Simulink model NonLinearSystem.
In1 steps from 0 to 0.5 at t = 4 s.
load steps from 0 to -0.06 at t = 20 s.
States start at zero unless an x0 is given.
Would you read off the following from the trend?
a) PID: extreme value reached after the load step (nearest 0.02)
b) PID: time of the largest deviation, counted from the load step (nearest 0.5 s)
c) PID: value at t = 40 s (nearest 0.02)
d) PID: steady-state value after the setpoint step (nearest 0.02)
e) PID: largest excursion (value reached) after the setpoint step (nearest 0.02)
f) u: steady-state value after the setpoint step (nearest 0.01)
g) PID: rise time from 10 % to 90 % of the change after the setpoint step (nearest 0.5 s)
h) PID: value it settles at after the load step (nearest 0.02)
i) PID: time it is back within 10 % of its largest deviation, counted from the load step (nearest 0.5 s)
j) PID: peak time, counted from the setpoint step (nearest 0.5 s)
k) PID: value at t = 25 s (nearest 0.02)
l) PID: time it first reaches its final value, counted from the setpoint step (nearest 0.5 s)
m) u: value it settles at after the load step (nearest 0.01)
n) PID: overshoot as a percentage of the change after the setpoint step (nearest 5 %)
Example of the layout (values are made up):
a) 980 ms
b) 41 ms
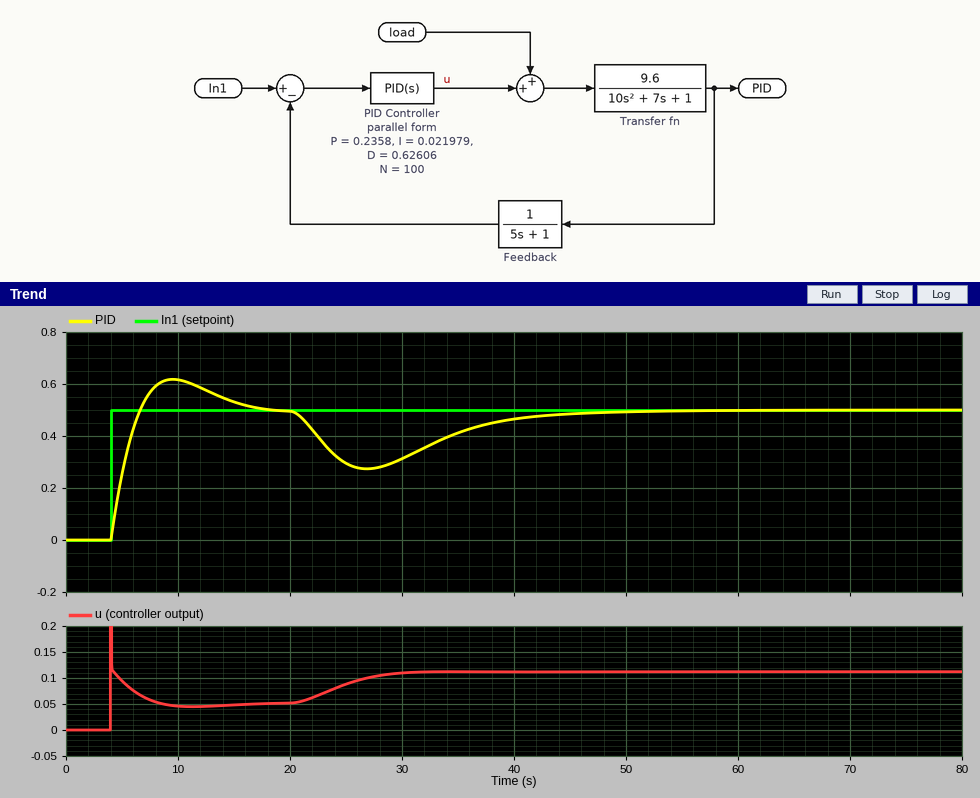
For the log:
a) 0.28
b) 7.0 s
c) 0.46
d) 0.50
e) 0.62
f) 0.05
g) 2.0 s
h) 0.50
i) 22.5 s
j) 5.5 s
k) 0.30
l) 2.5 s
m) 0.11
n) 25 %
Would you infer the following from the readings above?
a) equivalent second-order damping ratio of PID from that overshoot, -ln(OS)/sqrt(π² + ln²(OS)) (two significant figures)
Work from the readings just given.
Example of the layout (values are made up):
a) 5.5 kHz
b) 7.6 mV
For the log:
a) 0.40
